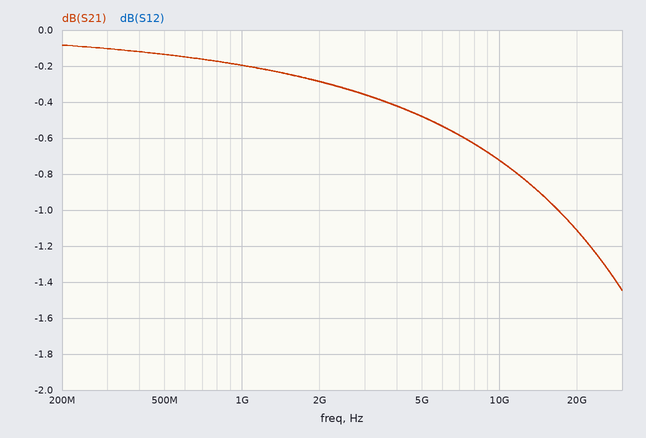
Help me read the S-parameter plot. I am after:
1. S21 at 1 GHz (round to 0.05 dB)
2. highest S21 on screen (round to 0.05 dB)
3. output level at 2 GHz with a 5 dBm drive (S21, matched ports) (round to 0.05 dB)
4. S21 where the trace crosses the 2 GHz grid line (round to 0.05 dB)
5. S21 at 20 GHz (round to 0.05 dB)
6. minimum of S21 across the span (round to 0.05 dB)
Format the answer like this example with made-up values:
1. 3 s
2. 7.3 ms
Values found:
1. -0.20 dB
2. -0.10 dB
3. 4.70 dBm
4. -0.30 dB
5. -1.10 dB
6. -1.45 dB
